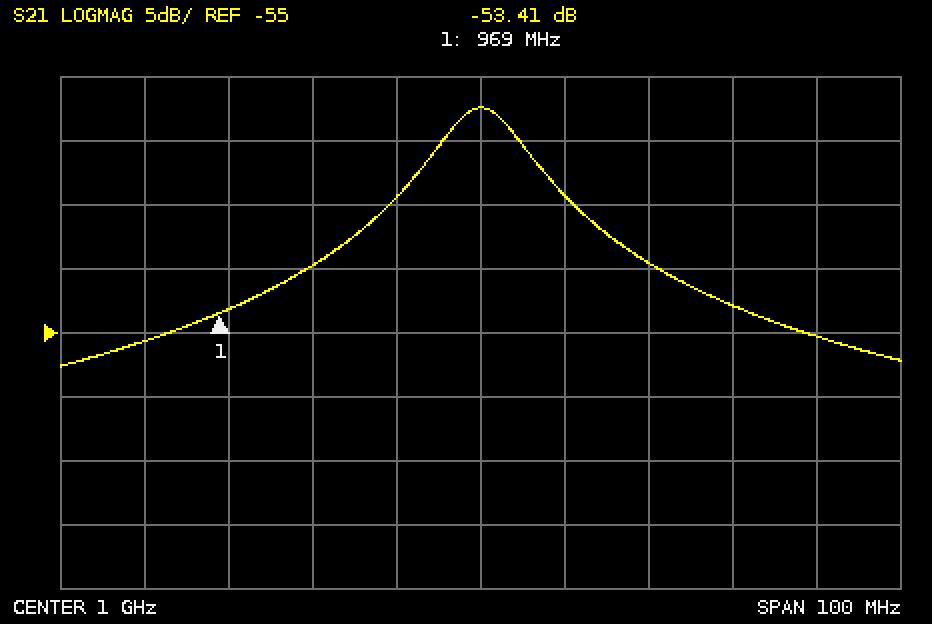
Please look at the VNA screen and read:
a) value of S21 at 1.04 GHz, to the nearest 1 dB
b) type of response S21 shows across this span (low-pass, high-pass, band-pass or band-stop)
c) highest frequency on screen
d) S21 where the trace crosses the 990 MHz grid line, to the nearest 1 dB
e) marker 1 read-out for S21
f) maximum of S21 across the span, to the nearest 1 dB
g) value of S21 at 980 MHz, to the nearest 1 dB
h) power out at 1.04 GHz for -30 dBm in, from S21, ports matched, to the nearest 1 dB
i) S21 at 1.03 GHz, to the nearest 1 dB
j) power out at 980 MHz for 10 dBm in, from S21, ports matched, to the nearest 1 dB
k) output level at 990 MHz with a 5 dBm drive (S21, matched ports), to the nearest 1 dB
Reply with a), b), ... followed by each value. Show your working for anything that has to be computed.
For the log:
a) -55 dB
b) band-pass
c) 1.05 GHz
d) -44 dB
e) -53.41 dB
f) -37 dB
g) -50 dB
h) -30 dBm + (-55 dB) = -85 dBm
i) -53 dB
j) 10 dBm + (-50 dB) = -40 dBm
k) 5 dBm + (-44 dB) = -39 dBm
